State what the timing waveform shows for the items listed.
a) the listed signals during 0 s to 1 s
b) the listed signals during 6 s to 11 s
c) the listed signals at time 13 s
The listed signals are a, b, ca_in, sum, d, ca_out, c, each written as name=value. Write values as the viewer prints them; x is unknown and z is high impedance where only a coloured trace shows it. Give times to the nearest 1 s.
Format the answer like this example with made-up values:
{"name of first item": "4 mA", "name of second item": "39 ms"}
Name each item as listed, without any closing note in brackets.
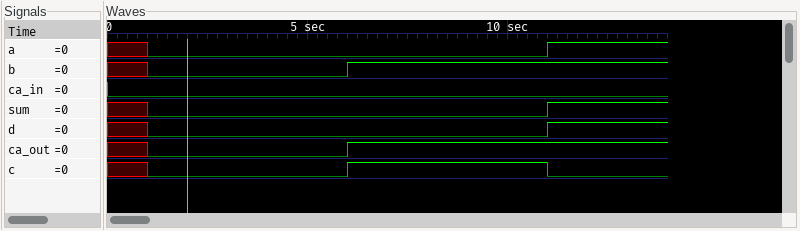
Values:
{"the listed signals during 0 s to 1 s": "a=x, b=x, ca_in=0, sum=x, d=x, ca_out=x, c=x", "the listed signals during 6 s to 11 s": "a=0, b=1, ca_in=0, sum=0, d=0, ca_out=1, c=1", "the listed signals at time 13 s": "a=1, b=1, ca_in=0, sum=1, d=1, ca_out=1, c=0"}
